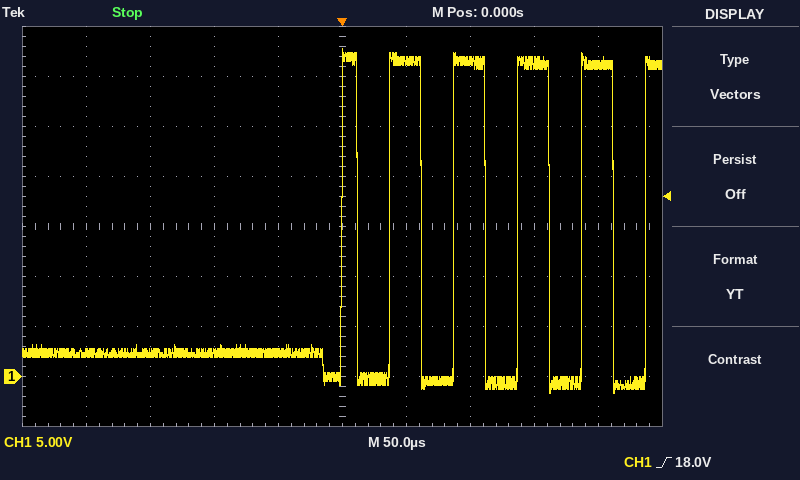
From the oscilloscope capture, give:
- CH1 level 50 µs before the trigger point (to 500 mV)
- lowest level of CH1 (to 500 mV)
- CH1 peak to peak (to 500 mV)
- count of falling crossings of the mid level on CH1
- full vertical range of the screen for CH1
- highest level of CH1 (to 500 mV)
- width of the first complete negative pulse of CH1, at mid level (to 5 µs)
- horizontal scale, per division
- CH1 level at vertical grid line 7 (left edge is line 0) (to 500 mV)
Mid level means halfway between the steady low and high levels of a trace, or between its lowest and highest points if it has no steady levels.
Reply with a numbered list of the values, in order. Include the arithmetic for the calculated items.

1. 2.5 V
2. -1.5 V
3. 33.0 V − (-1.5 V) = 34.5 V
4. 5
5. 40 V
6. 33.0 V
7. 25 µs
8. 50 µs
9. 31.5 V
